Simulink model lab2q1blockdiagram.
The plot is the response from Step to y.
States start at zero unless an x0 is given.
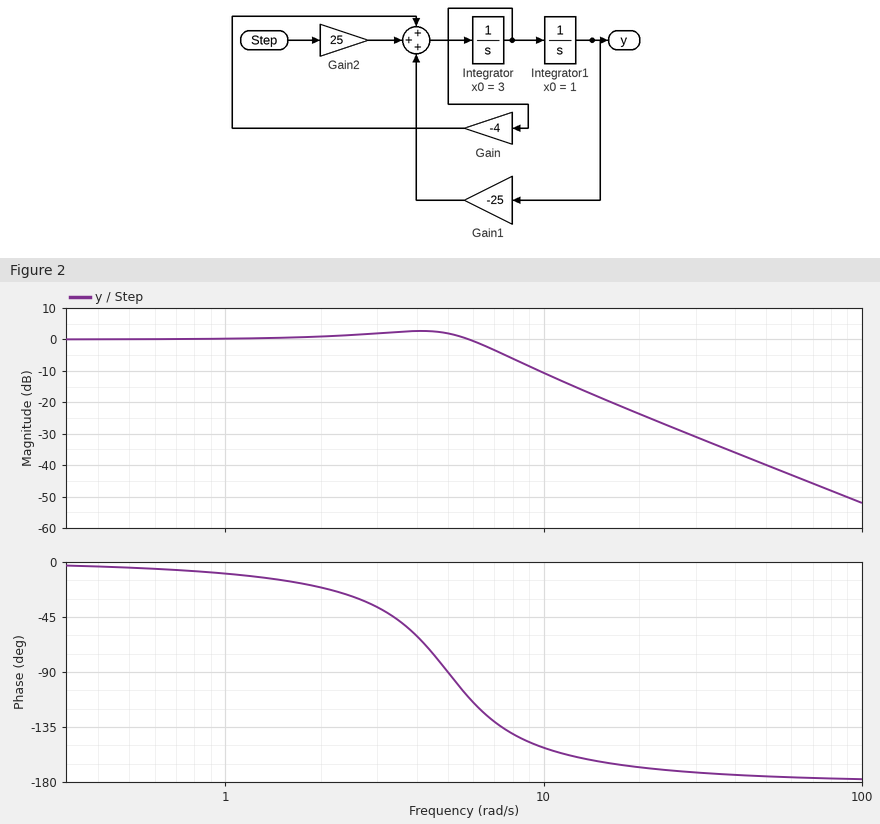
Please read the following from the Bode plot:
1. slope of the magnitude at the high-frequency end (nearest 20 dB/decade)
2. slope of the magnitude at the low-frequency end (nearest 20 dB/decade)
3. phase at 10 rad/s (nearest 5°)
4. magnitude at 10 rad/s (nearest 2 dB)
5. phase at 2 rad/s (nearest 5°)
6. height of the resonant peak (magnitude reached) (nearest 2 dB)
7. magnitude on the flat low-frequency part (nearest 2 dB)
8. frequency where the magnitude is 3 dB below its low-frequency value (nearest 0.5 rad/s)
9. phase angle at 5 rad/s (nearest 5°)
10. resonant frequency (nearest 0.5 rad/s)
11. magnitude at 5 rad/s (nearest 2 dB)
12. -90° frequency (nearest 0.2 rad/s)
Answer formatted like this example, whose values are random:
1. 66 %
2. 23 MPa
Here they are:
1. -40 dB/decade
2. 0 dB/decade
3. -150°
4. -10 dB
5. -20°
6. 2 dB
7. 0 dB
8. 7.0 rad/s
9. -90°
10. 4.0 rad/s
11. 2 dB
12. 5.0 rad/s
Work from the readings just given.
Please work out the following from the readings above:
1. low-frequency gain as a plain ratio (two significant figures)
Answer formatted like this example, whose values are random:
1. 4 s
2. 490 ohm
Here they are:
1. 1.0
